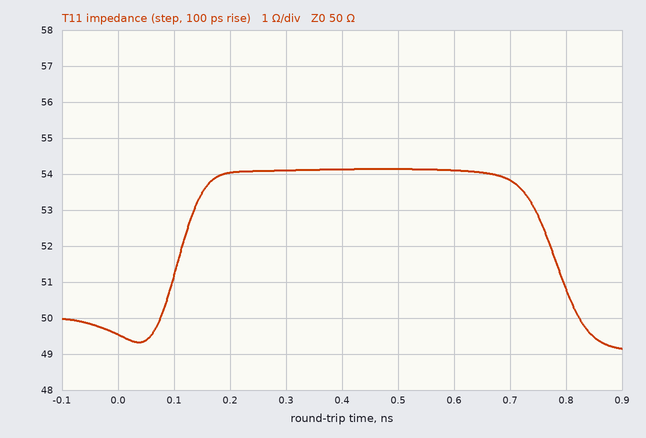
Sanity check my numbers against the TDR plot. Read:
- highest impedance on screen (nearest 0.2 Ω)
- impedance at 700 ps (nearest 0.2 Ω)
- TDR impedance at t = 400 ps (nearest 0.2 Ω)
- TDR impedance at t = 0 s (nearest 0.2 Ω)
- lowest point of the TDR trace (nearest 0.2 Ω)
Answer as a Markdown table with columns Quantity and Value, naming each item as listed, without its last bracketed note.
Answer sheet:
| Quantity | Value |
|---|---|
| highest impedance on screen | 54.2 Ω |
| impedance at 700 ps | 53.8 Ω |
| TDR impedance at t = 400 ps | 54.2 Ω |
| TDR impedance at t = 0 s | 49.6 Ω |
| lowest point of the TDR trace | 49.2 Ω |
